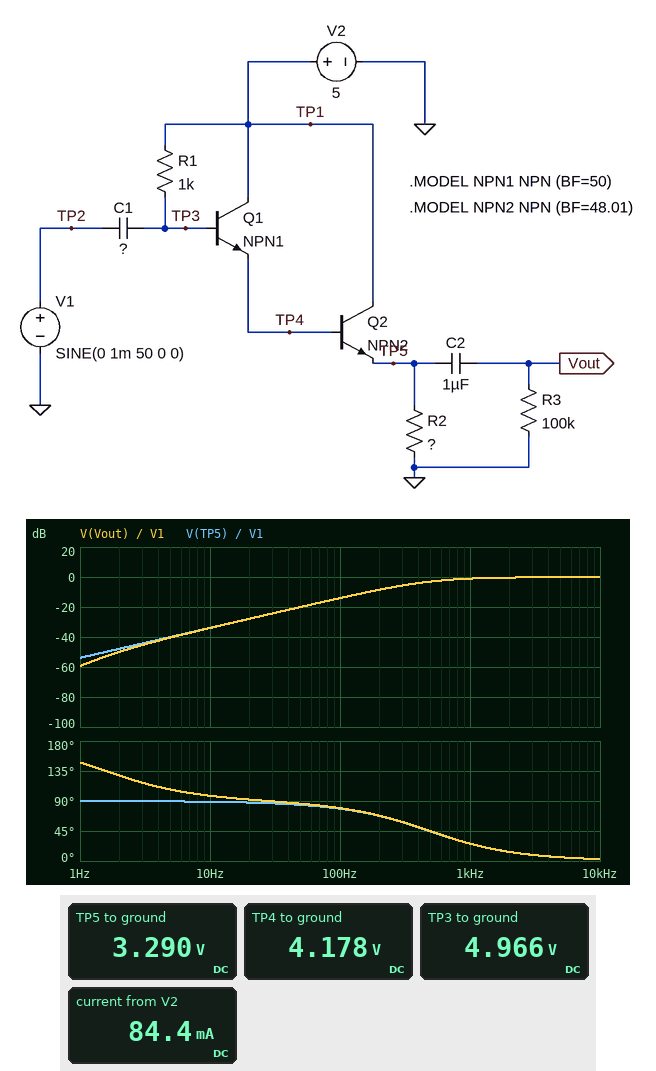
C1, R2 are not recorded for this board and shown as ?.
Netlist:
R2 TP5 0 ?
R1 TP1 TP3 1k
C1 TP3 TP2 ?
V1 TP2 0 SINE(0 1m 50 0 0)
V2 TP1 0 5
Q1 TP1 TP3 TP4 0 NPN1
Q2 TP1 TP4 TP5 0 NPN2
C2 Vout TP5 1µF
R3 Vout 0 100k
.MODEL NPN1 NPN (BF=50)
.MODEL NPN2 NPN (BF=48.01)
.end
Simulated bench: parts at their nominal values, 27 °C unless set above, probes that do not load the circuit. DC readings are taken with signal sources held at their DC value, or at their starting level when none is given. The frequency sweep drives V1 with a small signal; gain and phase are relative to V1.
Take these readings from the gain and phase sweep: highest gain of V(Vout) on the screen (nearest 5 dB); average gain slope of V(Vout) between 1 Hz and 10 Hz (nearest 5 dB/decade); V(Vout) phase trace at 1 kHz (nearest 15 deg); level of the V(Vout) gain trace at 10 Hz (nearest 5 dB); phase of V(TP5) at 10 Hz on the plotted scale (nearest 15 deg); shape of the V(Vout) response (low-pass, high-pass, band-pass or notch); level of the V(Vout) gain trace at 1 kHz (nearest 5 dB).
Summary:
0 dB
25 dB/decade
30 deg
-35 dB
90 deg
high-pass
0 dB
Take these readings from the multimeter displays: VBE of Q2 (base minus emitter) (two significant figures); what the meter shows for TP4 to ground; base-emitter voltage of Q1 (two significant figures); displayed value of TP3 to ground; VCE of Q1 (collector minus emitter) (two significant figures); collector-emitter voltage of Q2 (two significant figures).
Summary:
890 mV
4.178 V
790 mV
4.966 V
820 mV
1.7 V
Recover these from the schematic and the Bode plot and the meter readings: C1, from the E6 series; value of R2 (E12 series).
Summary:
330 nF
39 Ω
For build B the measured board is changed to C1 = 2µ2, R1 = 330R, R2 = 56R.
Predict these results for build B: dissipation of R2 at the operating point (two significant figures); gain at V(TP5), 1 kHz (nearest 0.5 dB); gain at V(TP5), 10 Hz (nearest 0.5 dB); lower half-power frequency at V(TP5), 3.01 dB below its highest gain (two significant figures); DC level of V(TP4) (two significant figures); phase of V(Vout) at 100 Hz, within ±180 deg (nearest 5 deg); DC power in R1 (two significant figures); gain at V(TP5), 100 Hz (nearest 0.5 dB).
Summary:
200 mW
-0.5 dB
-27.0 dB
220 Hz
4.2 V
65 deg
190 nW
-8.0 dB
